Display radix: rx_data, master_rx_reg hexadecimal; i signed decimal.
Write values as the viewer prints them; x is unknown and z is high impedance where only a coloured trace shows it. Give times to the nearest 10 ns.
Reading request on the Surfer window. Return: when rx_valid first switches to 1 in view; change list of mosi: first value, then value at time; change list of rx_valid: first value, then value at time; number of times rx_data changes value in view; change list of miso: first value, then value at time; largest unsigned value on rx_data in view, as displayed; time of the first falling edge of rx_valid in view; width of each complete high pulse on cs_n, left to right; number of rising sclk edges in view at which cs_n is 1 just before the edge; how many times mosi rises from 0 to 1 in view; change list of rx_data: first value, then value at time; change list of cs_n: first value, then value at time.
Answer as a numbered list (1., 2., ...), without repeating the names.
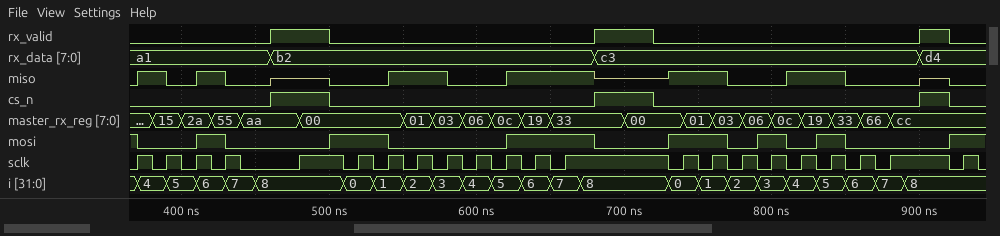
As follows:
1. 460 ns
2. 1, 0 at 370 ns, 1 at 410 ns, 0 at 430 ns, 1 at 500 ns, 0 at 540 ns, 1 at 620 ns, 0 at 680 ns, 1 at 730 ns, 0 at 770 ns, 1 at 790 ns, 0 at 810 ns, 1 at 830 ns, 0 at 850 ns, 1 at 920 ns
3. 0, 1 at 460 ns, 0 at 500 ns, 1 at 680 ns, 0 at 720 ns, 1 at 900 ns, 0 at 920 ns
4. 3
5. 0, 1 at 370 ns, 0 at 390 ns, 1 at 410 ns, 0 at 430 ns, z at 460 ns, 0 at 500 ns, 1 at 540 ns, 0 at 580 ns, 1 at 620 ns, z at 680 ns, 1 at 730 ns, 0 at 770 ns, 1 at 810 ns, 0 at 850 ns, z at 900 ns, 0 at 920 ns
6. d4
7. 500 ns
8. 40 ns, 40 ns, 20 ns
9. 1
10. 7
11. a1, b2 at 460 ns, c3 at 680 ns, d4 at 900 ns
12. 0, 1 at 460 ns, 0 at 500 ns, 1 at 680 ns, 0 at 720 ns, 1 at 900 ns, 0 at 920 ns
